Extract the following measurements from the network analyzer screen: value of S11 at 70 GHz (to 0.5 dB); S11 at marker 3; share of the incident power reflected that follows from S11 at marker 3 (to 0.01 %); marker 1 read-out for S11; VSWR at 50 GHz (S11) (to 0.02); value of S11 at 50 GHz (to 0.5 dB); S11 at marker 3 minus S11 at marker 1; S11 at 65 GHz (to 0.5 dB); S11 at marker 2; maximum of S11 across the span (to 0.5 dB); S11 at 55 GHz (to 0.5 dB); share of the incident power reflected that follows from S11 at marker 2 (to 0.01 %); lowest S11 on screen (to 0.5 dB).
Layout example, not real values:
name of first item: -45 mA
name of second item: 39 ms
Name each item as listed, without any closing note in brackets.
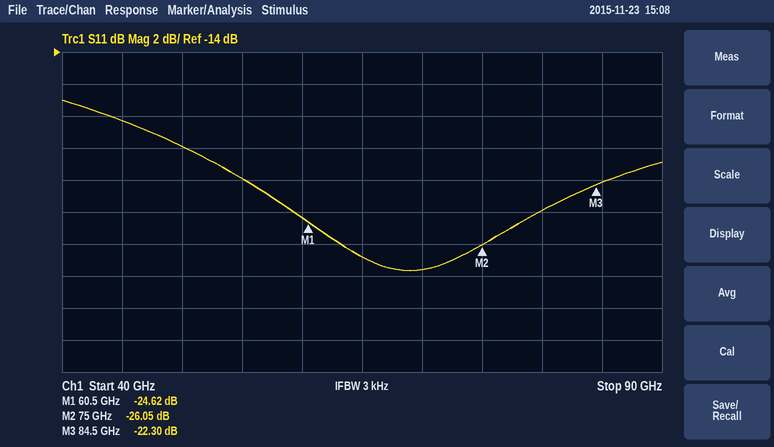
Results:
value of S11 at 70 GHz: -27.5 dB
S11 at marker 3: -22.30 dB
share of the incident power reflected that follows from S11 at marker 3: 0.59 %
marker 1 read-out for S11: -24.62 dB
VSWR at 50 GHz (S11): 1.22
value of S11 at 50 GHz: -20.0 dB
S11 at marker 3 minus S11 at marker 1: 2.32 dB
S11 at 65 GHz: -27.0 dB
S11 at marker 2: -26.05 dB
maximum of S11 across the span: -17.0 dB
S11 at 55 GHz: -22.0 dB
share of the incident power reflected that follows from S11 at marker 2: 0.25 %
lowest S11 on screen: -27.5 dB
